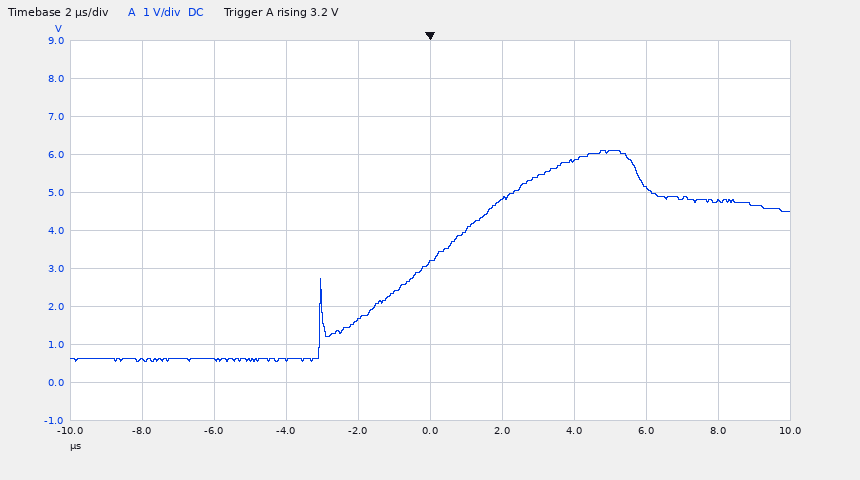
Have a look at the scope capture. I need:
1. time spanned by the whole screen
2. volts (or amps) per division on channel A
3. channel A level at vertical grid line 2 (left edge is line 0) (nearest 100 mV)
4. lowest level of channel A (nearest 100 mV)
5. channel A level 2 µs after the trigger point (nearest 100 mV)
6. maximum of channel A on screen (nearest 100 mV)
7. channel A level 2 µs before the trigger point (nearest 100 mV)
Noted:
20 µs
1 V
600 mV
600 mV
4.8 V
6.1 V
1.7 V
